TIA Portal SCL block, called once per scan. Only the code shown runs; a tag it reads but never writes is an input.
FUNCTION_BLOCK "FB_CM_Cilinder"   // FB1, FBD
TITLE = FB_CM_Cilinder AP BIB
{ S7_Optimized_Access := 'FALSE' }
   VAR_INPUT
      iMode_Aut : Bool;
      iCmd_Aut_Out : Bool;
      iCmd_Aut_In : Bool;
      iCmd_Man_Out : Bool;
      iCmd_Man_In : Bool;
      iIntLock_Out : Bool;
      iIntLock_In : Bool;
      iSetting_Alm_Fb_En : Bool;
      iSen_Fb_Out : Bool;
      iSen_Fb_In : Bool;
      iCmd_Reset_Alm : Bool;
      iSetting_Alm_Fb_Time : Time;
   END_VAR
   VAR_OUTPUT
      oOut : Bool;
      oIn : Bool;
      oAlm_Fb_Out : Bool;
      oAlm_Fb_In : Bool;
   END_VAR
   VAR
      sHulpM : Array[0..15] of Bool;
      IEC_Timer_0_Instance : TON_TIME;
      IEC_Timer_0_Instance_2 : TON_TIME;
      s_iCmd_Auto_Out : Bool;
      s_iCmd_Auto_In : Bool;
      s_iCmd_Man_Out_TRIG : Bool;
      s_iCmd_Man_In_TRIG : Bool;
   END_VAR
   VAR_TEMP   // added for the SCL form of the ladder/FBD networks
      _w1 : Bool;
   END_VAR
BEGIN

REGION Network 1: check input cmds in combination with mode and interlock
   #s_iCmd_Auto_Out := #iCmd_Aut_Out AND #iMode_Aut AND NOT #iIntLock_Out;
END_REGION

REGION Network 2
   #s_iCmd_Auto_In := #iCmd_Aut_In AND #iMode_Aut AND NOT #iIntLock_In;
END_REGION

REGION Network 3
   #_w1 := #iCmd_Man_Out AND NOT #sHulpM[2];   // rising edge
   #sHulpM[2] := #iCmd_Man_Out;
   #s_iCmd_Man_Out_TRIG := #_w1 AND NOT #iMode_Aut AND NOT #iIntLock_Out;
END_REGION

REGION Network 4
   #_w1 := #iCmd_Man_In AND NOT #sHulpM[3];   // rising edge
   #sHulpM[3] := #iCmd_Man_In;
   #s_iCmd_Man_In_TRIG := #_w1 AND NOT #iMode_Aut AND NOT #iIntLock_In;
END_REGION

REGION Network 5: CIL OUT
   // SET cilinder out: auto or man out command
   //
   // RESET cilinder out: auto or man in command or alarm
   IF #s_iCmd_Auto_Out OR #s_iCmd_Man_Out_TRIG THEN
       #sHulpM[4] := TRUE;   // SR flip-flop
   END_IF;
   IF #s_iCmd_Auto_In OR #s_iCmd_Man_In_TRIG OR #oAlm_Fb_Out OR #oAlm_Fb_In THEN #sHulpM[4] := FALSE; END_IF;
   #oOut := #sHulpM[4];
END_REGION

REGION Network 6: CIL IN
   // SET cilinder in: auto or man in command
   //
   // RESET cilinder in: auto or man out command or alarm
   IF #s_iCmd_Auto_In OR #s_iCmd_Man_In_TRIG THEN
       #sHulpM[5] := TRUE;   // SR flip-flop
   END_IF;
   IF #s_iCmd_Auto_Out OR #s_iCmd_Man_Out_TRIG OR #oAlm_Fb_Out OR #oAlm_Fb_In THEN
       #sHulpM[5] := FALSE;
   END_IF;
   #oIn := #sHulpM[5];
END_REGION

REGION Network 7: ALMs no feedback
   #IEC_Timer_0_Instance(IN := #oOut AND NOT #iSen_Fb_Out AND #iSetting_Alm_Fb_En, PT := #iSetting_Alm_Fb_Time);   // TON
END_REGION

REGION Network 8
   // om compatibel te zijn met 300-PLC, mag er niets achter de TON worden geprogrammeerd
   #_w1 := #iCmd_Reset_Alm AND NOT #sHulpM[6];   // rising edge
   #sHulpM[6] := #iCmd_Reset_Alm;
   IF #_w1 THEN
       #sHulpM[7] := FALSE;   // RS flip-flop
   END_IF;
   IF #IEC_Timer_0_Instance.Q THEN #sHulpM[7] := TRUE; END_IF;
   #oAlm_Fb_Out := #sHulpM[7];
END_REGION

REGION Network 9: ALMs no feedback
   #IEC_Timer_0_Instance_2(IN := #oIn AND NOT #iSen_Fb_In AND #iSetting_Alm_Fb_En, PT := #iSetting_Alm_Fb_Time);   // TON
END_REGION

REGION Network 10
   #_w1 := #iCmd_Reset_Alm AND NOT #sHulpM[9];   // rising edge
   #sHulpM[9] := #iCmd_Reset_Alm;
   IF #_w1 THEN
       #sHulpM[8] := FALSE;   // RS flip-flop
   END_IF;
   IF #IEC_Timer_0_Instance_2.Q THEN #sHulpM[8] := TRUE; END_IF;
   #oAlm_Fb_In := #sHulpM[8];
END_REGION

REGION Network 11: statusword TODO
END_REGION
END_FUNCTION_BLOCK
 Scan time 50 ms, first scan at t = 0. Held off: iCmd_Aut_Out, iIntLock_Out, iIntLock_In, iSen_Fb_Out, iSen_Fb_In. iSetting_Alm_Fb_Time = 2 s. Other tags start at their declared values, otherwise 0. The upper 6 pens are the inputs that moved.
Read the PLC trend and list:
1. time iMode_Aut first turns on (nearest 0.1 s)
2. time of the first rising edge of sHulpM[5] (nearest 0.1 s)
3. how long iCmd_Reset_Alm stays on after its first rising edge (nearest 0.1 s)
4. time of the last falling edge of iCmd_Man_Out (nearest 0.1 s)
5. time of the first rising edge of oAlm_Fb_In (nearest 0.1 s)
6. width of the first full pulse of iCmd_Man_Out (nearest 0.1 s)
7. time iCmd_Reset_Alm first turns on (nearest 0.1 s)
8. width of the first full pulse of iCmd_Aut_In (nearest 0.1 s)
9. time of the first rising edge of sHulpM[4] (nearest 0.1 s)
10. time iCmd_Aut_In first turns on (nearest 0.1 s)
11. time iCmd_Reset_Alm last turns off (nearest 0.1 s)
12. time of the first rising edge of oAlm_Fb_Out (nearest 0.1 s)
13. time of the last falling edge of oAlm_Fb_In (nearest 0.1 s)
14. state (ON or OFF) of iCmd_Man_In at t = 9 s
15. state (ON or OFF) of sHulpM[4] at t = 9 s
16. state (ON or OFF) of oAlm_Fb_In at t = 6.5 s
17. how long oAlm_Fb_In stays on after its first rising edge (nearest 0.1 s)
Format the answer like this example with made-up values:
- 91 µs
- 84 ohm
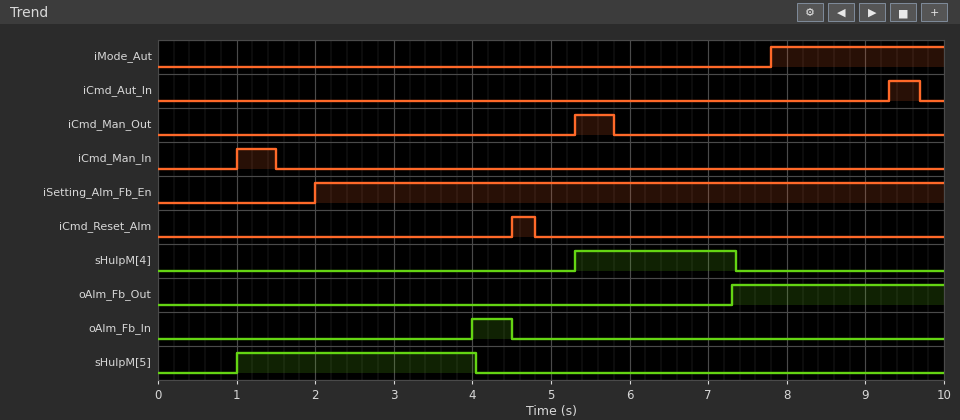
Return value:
- 7.8 s
- 1.0 s
- 0.3 s
- 5.8 s
- 4.0 s
- 0.5 s
- 4.5 s
- 0.4 s
- 5.3 s
- 9.3 s
- 4.8 s
- 7.3 s
- 4.5 s
- OFF
- OFF
- OFF
- 0.5 s
